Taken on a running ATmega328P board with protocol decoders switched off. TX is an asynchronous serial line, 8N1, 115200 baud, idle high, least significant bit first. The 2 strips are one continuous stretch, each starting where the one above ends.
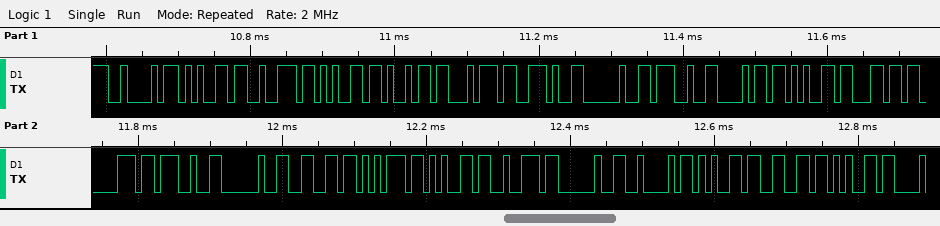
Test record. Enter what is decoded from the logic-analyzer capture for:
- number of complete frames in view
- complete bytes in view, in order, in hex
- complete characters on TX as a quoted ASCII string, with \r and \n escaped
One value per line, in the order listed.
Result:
24
42 65 72 65 69 74 2E 20 27 68 65 6C 70 27 20 66 75 65 72 20 42 65 66 65
"Bereit. 'help' fuer Befe"
